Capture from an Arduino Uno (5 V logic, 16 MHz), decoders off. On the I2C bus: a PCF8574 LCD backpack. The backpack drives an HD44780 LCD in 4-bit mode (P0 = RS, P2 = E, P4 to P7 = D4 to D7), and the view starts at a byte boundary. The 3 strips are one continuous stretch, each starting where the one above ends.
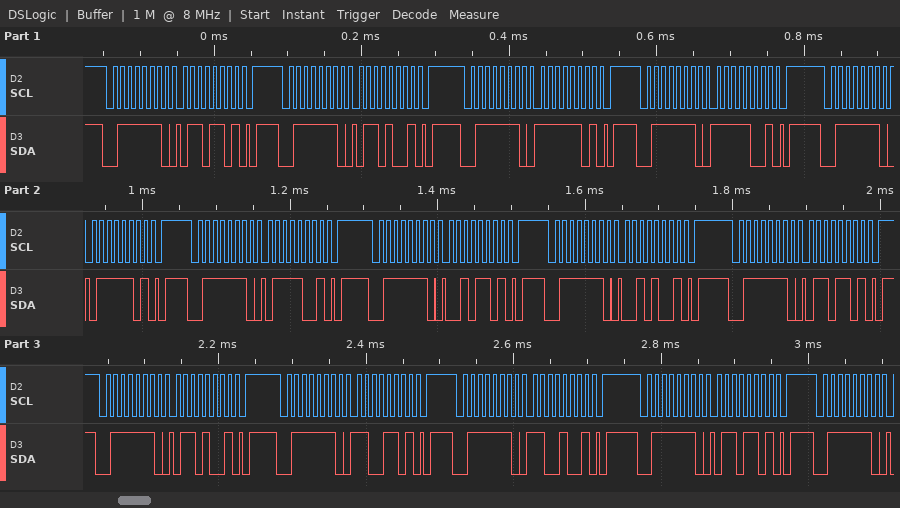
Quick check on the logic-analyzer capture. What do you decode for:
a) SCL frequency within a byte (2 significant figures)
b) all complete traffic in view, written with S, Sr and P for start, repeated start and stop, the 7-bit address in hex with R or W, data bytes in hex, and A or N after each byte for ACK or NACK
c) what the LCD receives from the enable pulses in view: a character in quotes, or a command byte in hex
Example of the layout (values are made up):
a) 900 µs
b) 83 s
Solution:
a) 100 kHz
b) S 3FW A 6D A P S 3FW A 69 A P S 3FW A FD A P S 3FW A F9 A P S 3FW A 7D A P S 3FW A 79 A P S 3FW A 2D A P S 3FW A 29 A P S 3FW A 6D A P S 3FW A 69 A P S 3FW A CD A P S 3FW A C9 A P S 3FW A 6D A P S 3FW A
c) 'o' 'r' 'l'
